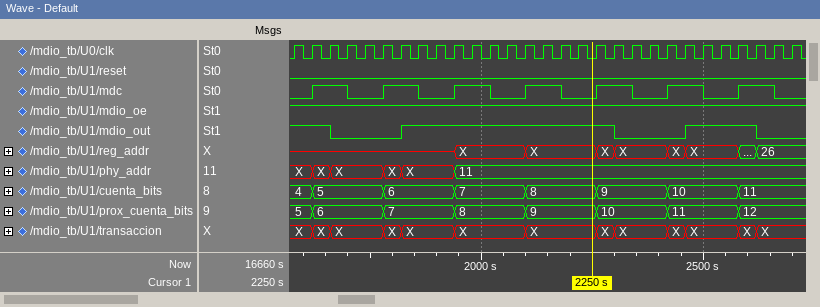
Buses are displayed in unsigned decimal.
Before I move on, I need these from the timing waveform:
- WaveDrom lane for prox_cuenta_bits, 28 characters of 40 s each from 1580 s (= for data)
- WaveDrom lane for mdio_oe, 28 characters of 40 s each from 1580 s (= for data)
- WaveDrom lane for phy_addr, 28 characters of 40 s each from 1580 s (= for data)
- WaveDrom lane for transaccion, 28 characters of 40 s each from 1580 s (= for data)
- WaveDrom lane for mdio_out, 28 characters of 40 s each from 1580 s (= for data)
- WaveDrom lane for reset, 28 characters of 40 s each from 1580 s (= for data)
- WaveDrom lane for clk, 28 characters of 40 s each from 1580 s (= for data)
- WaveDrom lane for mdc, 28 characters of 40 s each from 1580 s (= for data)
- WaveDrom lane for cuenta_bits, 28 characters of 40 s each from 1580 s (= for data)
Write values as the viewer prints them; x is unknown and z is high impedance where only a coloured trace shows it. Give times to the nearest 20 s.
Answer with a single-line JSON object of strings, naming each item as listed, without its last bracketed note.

{"WaveDrom lane for prox_cuenta_bits, 28 characters of 40 s each from 1580 s": "{name: 'prox_cuenta_bits', wave: '==...=...=...=...=...=...=..', data: '5 6 7 8 9 10 11 12'}", "WaveDrom lane for mdio_oe, 28 characters of 40 s each from 1580 s": "{name: 'mdio_oe', wave: '1...........................'}", "WaveDrom lane for phy_addr, 28 characters of 40 s each from 1580 s": "{name: 'phy_addr', wave: '===..==..=..................', data: 'X X X X X 11'}", "WaveDrom lane for transaccion, 28 characters of 40 s each from 1580 s": "{name: 'transaccion', wave: '===..==..=...=...==..==..==.', data: 'X X X X X X X X X X X X X'}", "WaveDrom lane for mdio_out, 28 characters of 40 s each from 1580 s": "{name: 'mdio_out', wave: '1.0...1...........0...1...0.'}", "WaveDrom lane for reset, 28 characters of 40 s each from 1580 s": "{name: 'reset', wave: '0...........................'}", "WaveDrom lane for clk, 28 characters of 40 s each from 1580 s": "{name: 'clk', wave: 'p...........................'}", "WaveDrom lane for mdc, 28 characters of 40 s each from 1580 s": "{name: 'mdc', wave: '01.0.1.0.1.0.1.0.1.0.1.0.1.0'}", "WaveDrom lane for cuenta_bits, 28 characters of 40 s each from 1580 s": "{name: 'cuenta_bits', wave: '==...=...=...=...=...=...=..', data: '4 5 6 7 8 9 10 11'}"}
